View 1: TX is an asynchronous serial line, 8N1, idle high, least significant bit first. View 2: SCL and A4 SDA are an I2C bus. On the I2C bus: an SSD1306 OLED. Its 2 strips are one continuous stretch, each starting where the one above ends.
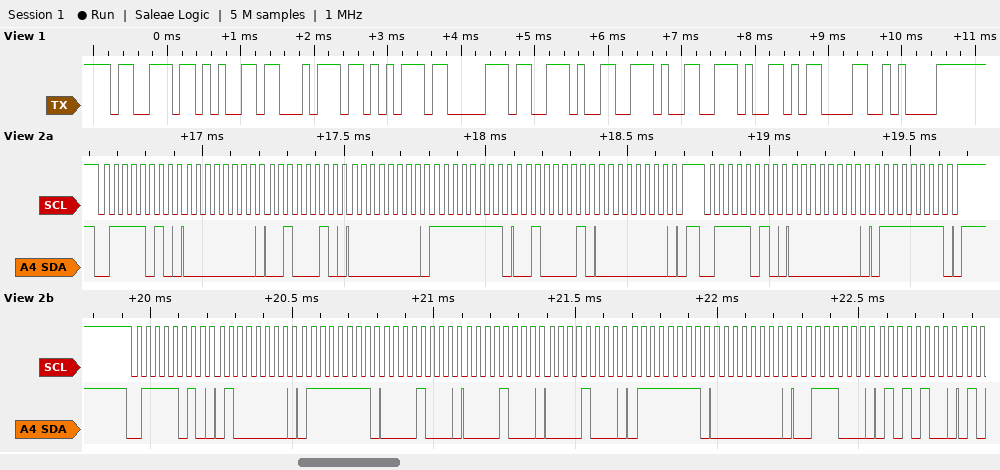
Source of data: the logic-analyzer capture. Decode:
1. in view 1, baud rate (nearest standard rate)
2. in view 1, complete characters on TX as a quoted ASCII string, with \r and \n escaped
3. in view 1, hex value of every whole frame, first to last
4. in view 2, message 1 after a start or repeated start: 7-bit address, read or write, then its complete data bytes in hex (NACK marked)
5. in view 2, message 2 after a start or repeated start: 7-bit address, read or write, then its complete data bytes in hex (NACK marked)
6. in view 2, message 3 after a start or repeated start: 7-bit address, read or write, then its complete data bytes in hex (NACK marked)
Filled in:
9600 baud
"setup...\r\n"
73 65 74 75 70 2E 2E 2E 0D 0A
0x3D write: 00 22 00 FF 21 00
0x3D write: 00 7F
0x3D write: 40 7F 08 08 08 7F 00 38 54
